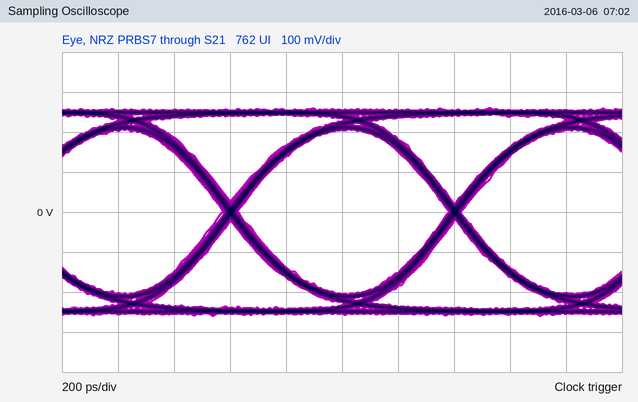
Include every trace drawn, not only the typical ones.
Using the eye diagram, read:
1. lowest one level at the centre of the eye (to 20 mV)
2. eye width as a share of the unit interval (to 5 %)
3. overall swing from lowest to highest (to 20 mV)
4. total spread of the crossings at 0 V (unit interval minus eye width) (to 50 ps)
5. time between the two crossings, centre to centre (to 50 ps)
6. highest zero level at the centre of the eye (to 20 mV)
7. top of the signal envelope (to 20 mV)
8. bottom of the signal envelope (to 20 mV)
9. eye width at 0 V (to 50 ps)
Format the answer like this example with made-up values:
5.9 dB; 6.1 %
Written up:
200 mV; 95 %; 520 mV; 50 ps; 800 ps; -200 mV; 260 mV; -260 mV; 750 ps
